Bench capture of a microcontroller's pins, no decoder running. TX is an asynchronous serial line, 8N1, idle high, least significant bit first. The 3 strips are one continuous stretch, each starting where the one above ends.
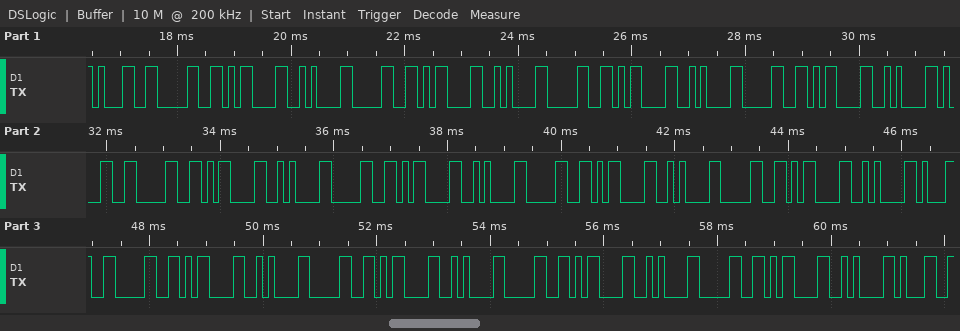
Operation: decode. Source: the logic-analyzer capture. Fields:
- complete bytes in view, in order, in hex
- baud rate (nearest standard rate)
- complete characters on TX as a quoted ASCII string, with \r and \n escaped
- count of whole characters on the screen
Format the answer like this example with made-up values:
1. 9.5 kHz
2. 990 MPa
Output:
1. 31 30 0D 0A 30 0D 0A 30 0D 0A 30 0D 0A 31 30 0D 0A 30 0D 0A 30 0D 0A 30 0D 0A 31 30 0D 0A 30 0D 0A 30 0D 0A 30 0D 0A 31
2. 9600 baud
3. "10\r\n0\r\n0\r\n0\r\n10\r\n0\r\n0\r\n0\r\n10\r\n0\r\n0\r\n0\r\n1"
4. 40
